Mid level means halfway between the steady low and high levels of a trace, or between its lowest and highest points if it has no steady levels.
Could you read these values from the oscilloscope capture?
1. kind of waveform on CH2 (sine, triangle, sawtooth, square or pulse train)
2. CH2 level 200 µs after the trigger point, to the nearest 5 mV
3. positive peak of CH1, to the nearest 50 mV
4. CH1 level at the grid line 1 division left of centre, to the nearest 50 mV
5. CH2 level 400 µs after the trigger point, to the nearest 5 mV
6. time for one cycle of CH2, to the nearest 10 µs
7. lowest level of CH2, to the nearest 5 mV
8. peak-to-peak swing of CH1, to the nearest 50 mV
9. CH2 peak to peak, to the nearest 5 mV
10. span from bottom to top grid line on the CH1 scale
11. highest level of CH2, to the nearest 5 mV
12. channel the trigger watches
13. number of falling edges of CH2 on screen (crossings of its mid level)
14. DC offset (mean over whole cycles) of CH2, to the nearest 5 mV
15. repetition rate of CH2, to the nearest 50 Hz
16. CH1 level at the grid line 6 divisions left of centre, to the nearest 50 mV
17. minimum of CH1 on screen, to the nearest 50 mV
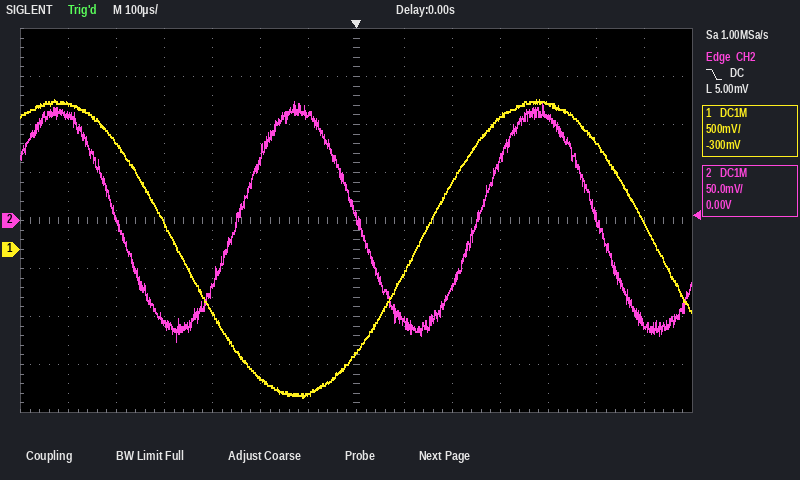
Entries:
sine
-70 mV
1.55 V
-1.50 V
105 mV
500 µs
-125 mV
3.10 V
250 mV
4 V
125 mV
CH2
3
0 mV
2.00 kHz
1.50 V
-1.55 V
